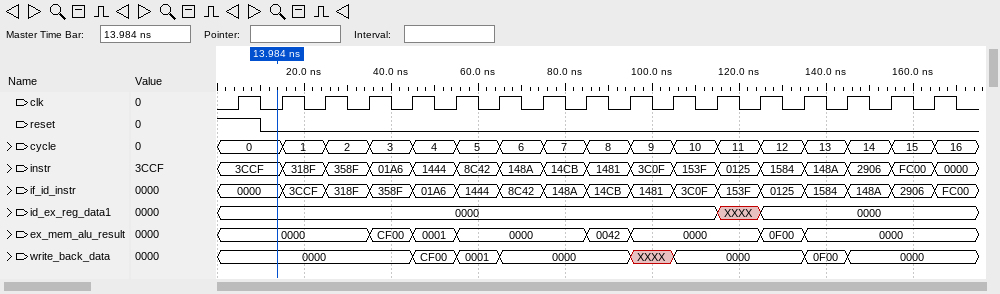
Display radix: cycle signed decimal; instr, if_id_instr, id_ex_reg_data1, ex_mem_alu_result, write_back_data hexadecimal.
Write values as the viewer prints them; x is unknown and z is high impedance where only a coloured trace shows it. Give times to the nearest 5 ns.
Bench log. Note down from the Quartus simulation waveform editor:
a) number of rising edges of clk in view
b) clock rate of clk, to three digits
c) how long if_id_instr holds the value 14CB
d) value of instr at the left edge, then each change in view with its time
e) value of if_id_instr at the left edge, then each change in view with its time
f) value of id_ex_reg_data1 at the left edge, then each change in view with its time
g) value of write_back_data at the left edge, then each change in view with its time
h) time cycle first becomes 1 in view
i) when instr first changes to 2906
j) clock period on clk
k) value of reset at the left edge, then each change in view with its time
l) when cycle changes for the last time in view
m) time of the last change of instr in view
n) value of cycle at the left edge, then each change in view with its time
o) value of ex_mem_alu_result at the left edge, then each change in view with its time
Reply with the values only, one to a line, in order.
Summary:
17
100 MHz
10 ns
3CCF, 318F at 15 ns, 358F at 25 ns, 01A6 at 35 ns, 1444 at 45 ns, 8C42 at 55 ns, 148A at 65 ns, 14CB at 75 ns, 1481 at 85 ns, 3C0F at 95 ns, 153F at 105 ns, 0125 at 115 ns, 1584 at 125 ns, 148A at 135 ns, 2906 at 145 ns, FC00 at 155 ns, 0000 at 165 ns
0000, 3CCF at 15 ns, 318F at 25 ns, 358F at 35 ns, 01A6 at 45 ns, 1444 at 55 ns, 8C42 at 65 ns, 148A at 75 ns, 14CB at 85 ns, 1481 at 95 ns, 3C0F at 105 ns, 153F at 115 ns, 0125 at 125 ns, 1584 at 135 ns, 148A at 145 ns, 2906 at 155 ns, FC00 at 165 ns
0000, XXXX at 115 ns, 0000 at 125 ns
0000, CF00 at 45 ns, 0001 at 55 ns, 0000 at 65 ns, XXXX at 95 ns, 0000 at 105 ns, 0F00 at 135 ns, 0000 at 145 ns
15 ns
145 ns
10 ns
1, 0 at 10 ns
165 ns
165 ns
0, 1 at 15 ns, 2 at 25 ns, 3 at 35 ns, 4 at 45 ns, 5 at 55 ns, 6 at 65 ns, 7 at 75 ns, 8 at 85 ns, 9 at 95 ns, 10 at 105 ns, 11 at 115 ns, 12 at 125 ns, 13 at 135 ns, 14 at 145 ns, 15 at 155 ns, 16 at 165 ns
0000, CF00 at 35 ns, 0001 at 45 ns, 0000 at 55 ns, 0042 at 85 ns, 0000 at 95 ns, 0F00 at 125 ns, 0000 at 135 ns
